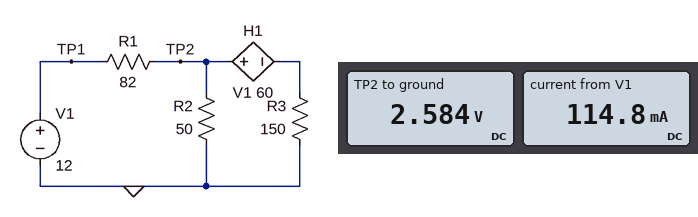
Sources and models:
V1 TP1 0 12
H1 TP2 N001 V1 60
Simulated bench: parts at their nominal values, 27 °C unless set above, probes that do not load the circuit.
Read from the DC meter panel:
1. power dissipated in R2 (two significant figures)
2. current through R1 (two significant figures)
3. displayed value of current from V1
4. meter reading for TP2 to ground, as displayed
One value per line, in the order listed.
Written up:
130 mW
110 mA
114.8 mA
2.584 V
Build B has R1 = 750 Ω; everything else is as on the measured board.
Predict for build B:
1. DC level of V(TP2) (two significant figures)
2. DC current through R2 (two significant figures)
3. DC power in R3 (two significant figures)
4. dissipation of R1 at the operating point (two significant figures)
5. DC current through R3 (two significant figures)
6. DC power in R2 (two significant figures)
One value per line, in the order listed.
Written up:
350 mV
7.0 mA
11 mW
180 mW
8.5 mA
2.4 mW
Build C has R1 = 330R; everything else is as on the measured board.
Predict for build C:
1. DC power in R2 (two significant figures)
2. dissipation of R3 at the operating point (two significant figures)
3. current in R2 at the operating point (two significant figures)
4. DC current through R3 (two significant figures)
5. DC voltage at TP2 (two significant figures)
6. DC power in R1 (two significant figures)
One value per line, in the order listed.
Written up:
12 mW
53 mW
15 mA
19 mA
770 mV
380 mW
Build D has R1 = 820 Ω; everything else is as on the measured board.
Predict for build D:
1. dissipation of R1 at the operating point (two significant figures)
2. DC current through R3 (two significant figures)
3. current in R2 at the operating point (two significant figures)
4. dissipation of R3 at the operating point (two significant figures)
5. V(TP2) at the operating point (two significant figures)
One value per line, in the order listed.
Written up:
170 mW
7.8 mA
6.4 mA
9.2 mW
320 mV
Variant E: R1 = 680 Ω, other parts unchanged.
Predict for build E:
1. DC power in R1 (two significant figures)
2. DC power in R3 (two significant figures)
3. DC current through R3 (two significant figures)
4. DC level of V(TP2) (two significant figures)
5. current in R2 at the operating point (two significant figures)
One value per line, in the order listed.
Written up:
200 mW
13 mW
9.4 mA
380 mV
7.7 mA
